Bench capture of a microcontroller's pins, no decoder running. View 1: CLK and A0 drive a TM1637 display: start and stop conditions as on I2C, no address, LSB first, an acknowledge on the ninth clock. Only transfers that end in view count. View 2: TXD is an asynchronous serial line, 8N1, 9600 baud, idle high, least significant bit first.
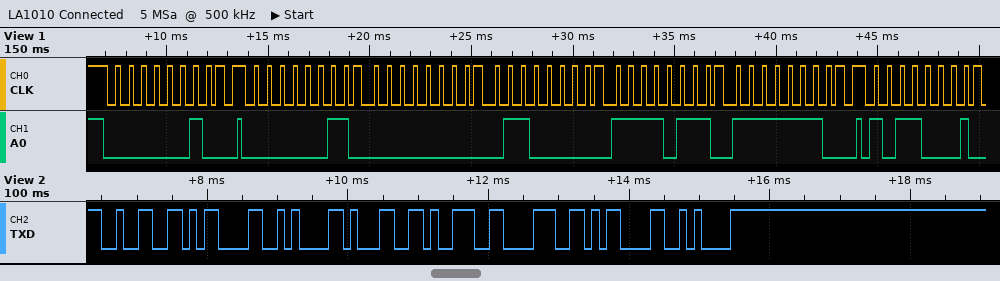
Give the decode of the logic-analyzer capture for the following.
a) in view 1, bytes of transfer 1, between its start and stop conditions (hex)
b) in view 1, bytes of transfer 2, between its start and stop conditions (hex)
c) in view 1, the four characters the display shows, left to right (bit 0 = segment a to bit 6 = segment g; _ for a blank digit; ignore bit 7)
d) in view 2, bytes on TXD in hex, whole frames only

40
C0 00 06 EF 7F
_198
0x32 0x0D 0x0A 0x31 0x39 0x38 0x0D 0x0A
